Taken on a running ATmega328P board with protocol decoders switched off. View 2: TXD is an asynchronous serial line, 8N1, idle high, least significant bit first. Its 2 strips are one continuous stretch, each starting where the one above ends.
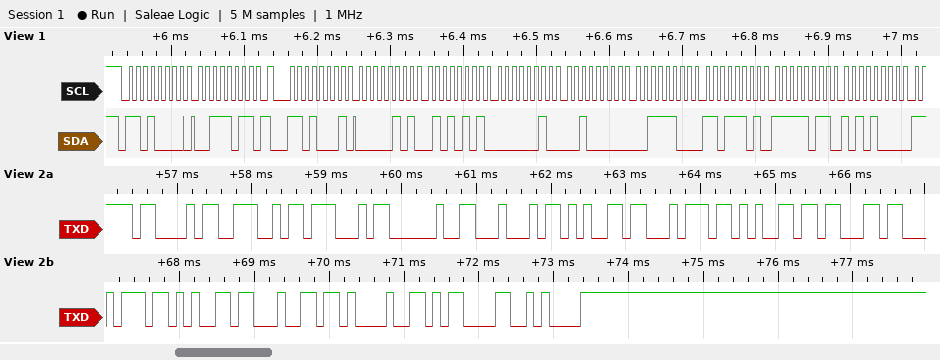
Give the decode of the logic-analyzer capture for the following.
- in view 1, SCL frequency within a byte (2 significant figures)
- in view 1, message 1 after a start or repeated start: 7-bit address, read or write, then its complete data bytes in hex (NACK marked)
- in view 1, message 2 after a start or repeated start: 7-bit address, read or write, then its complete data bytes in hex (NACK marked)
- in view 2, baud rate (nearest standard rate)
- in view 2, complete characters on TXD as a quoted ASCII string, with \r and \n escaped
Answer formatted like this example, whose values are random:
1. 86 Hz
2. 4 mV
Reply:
1. 100 kHz
2. 0x68 write: 3B
3. 0x68 read: 05 55 02 20 3C DD FB A8
4. 9600 baud
5. "CNG Detected!\r\n"
